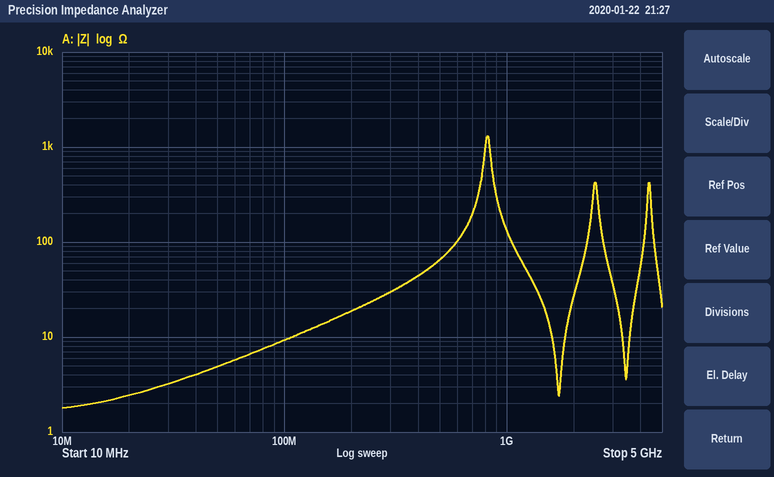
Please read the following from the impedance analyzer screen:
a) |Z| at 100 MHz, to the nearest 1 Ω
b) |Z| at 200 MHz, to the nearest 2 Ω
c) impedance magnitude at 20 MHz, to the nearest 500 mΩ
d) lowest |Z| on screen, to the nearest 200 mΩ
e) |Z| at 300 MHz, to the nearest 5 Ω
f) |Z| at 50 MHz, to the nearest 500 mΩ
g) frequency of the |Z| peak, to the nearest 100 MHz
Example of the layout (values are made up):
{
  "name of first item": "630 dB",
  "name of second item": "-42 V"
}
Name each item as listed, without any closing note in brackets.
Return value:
{
  "|Z| at 100 MHz, to the nearest 1 Ω": "9 Ω",
  "|Z| at 200 MHz, to the nearest 2 Ω": "18 Ω",
  "impedance magnitude at 20 MHz, to the nearest 500 mΩ": "2.5 Ω",
  "lowest |Z| on screen, to the nearest 200 mΩ": "1.8 Ω",
  "|Z| at 300 MHz, to the nearest 5 Ω": "30 Ω",
  "|Z| at 50 MHz, to the nearest 500 mΩ": "5.0 Ω",
  "frequency of the |Z| peak, to the nearest 100 MHz": "800 MHz"
}
